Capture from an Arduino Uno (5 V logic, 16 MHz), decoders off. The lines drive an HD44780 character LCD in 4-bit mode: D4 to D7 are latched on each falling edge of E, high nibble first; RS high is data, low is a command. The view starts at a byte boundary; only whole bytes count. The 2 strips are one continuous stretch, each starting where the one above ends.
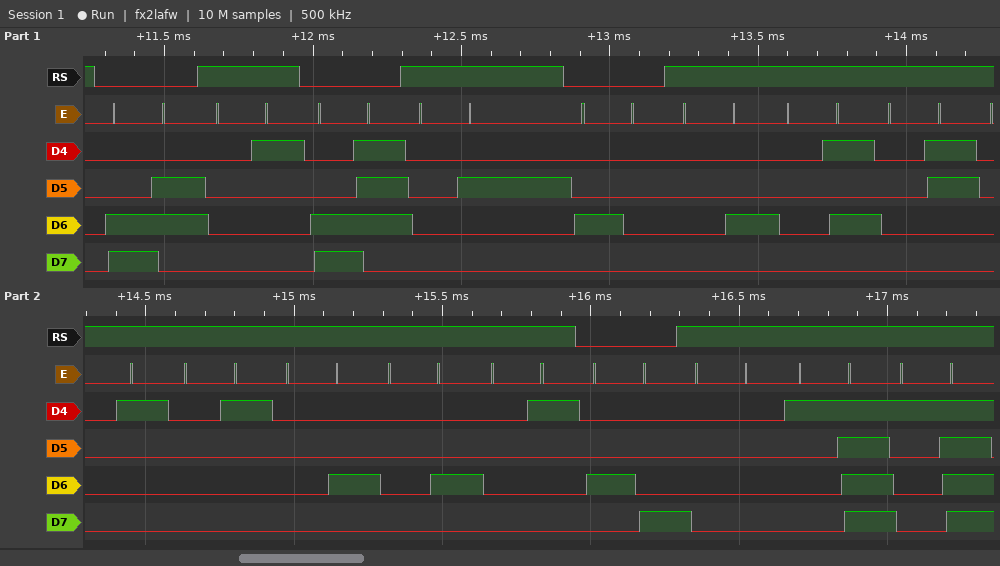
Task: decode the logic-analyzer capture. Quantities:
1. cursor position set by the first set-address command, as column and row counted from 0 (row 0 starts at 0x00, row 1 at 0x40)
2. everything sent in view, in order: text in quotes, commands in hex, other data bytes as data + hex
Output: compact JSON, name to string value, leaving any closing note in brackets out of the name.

{"cursor position set by the first set-address command, as column and row counted from 0": "column 6, row 1", "everything sent in view, in order: text in quotes, commands in hex, other data bytes as data + hex": "0xC6 data 01 0xC7 data 02 0x40 data 04 05 03 01 01 04 04 01 0x48 data 00 1F 1F"}
